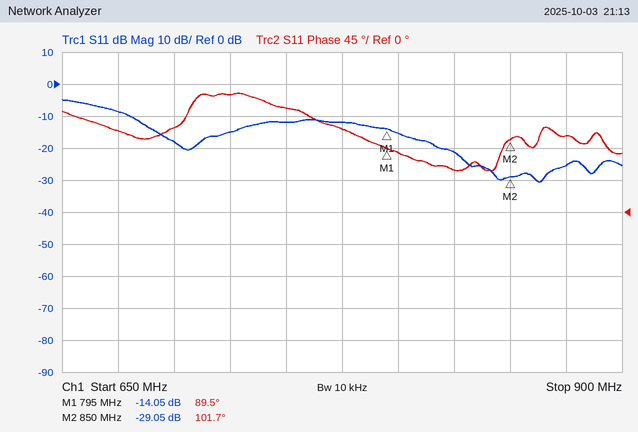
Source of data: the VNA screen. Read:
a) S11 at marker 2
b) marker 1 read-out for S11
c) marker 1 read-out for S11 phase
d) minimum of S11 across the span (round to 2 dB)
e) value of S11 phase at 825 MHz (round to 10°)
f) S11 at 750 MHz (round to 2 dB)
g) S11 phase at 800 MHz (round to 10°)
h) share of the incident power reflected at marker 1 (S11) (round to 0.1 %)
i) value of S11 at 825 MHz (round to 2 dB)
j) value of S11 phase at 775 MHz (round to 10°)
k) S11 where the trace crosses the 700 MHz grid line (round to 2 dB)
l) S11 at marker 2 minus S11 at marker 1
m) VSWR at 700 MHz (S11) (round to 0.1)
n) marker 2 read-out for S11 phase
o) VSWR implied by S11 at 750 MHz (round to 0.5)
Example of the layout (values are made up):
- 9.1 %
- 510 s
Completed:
- -29.05 dB
- -14.05 dB
- 89.5°
- -30 dB
- 60°
- -12 dB
- 80°
- 3.9 %
- -22 dB
- 120°
- -18 dB
- -15.00 dB
- 1.3
- 101.7°
- 1.5
